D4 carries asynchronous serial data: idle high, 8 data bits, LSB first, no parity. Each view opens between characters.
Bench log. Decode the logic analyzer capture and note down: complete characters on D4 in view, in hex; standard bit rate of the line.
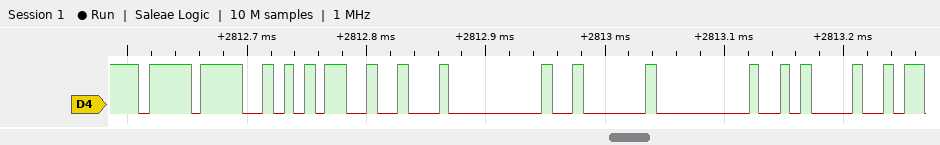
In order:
EF, AA, 12, 00, 02, 00, 0A
115200 baud
